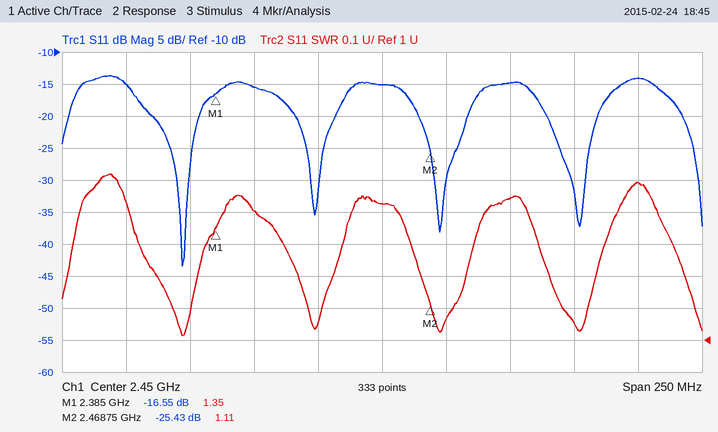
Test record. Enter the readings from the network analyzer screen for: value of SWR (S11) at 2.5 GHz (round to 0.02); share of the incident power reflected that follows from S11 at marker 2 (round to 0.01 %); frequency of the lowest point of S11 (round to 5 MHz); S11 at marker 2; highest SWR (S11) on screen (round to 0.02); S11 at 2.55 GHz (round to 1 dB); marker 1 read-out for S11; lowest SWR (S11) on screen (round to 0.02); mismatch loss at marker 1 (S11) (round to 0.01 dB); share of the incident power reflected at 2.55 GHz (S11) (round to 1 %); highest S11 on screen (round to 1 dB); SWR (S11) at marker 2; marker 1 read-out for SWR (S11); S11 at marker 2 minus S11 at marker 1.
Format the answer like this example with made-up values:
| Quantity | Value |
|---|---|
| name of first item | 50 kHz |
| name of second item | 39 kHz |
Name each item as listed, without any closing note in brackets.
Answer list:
| Quantity | Value |
|---|---|
| value of SWR (S11) at 2.5 GHz | 1.44 |
| share of the incident power reflected that follows from S11 at marker 2 | 0.29 % |
| frequency of the lowest point of S11 | 2.370 GHz |
| S11 at marker 2 | -25.43 dB |
| highest SWR (S11) on screen | 1.52 |
| S11 at 2.55 GHz | -14 dB |
| marker 1 read-out for S11 | -16.55 dB |
| lowest SWR (S11) on screen | 1.02 |
| mismatch loss at marker 1 (S11) | 0.10 dB |
| share of the incident power reflected at 2.55 GHz (S11) | 4 % |
| highest S11 on screen | -14 dB |
| SWR (S11) at marker 2 | 1.11 |
| marker 1 read-out for SWR | 1.35 |
| S11 at marker 2 minus S11 at marker 1 | -8.88 dB |
